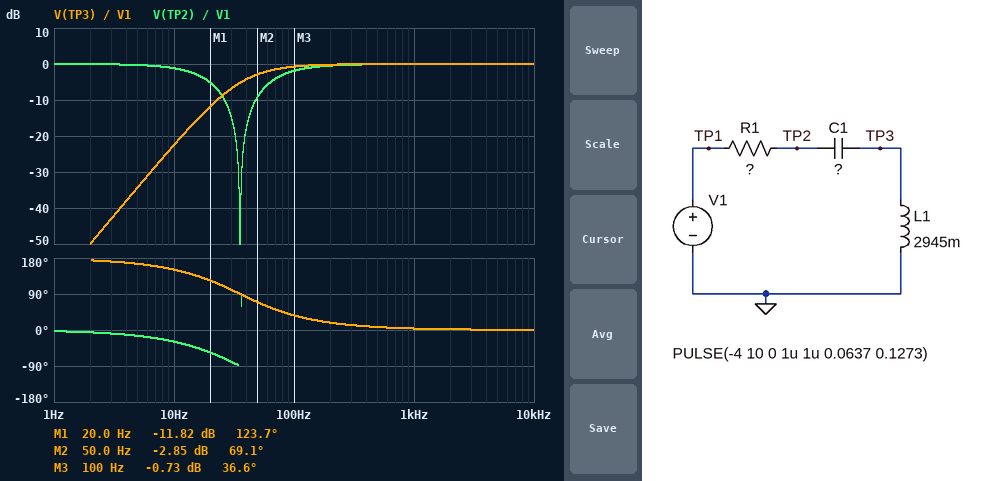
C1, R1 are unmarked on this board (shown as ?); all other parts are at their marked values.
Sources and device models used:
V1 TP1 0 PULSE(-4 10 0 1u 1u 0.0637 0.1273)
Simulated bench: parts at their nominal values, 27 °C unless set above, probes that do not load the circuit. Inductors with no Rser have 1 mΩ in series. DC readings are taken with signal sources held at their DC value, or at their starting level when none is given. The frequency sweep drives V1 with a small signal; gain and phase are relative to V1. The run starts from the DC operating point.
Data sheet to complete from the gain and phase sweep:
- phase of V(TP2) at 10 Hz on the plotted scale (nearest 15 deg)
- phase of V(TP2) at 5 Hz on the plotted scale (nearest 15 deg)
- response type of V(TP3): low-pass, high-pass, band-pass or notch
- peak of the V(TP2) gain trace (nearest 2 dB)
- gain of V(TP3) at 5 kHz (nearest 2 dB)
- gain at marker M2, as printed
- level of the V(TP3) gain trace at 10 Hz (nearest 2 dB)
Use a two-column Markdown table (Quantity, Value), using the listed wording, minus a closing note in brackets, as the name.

| Quantity | Value |
|---|---|
| phase of V(TP2) at 10 Hz on the plotted scale | -30 deg |
| phase of V(TP2) at 5 Hz on the plotted scale | -15 deg |
| response type of V(TP3): low-pass, high-pass, band-pass or notch | high-pass |
| peak of the V(TP2) gain trace | 0 dB |
| gain of V(TP3) at 5 kHz | 0 dB |
| gain at marker M2, as printed | -2.85 dB |
| level of the V(TP3) gain trace at 10 Hz | -22 dB |
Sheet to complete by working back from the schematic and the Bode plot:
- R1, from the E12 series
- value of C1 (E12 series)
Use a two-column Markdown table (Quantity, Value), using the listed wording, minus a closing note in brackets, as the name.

| Quantity | Value |
|---|---|
| R1, from the E12 series | 1.2 kΩ |
| value of C1 | 6.8 µF |
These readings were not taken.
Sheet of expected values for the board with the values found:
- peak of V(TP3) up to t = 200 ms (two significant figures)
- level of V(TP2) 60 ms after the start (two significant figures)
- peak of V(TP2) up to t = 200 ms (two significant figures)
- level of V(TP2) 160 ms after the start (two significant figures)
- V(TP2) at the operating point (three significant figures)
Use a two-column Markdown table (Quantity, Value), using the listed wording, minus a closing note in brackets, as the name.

| Quantity | Value |
|---|---|
| peak of V(TP3) up to t = 200 ms | 14 V |
| level of V(TP2) 60 ms after the start | 10 V |
| peak of V(TP2) up to t = 200 ms | 10 V |
| level of V(TP2) 160 ms after the start | 10 V |
| V(TP2) at the operating point | -4.00 V |
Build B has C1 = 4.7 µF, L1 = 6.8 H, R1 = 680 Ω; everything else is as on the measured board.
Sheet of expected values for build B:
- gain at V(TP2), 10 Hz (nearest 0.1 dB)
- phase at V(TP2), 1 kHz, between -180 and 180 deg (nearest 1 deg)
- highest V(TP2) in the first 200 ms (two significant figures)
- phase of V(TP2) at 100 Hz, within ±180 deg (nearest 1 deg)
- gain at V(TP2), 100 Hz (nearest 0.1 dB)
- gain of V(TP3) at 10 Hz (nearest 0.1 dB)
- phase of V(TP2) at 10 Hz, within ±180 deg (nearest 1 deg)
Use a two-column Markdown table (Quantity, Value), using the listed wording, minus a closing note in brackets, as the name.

| Quantity | Value |
|---|---|
| gain at V(TP2), 10 Hz | -0.2 dB |
| phase at V(TP2), 1 kHz, between -180 and 180 deg | 1 deg |
| highest V(TP2) in the first 200 ms | 12 V |
| phase of V(TP2) at 100 Hz, within ±180 deg | 10 deg |
| gain at V(TP2), 100 Hz | -0.1 dB |
| gain of V(TP3) at 10 Hz | -17.0 dB |
| phase of V(TP2) at 10 Hz, within ±180 deg | -13 deg |
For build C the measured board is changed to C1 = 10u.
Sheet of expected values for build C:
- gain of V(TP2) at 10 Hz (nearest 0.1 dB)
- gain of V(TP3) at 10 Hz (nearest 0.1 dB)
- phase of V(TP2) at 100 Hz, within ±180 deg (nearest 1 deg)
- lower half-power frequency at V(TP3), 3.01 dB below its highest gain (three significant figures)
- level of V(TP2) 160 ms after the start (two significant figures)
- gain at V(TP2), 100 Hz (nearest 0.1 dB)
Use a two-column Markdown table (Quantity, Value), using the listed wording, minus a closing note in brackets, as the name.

| Quantity | Value |
|---|---|
| gain of V(TP2) at 10 Hz | -2.4 dB |
| gain of V(TP3) at 10 Hz | -20.0 dB |
| phase of V(TP2) at 100 Hz, within ±180 deg | 35 deg |
| lower half-power frequency at V(TP3), 3.01 dB below its highest gain | 52.5 Hz |
| level of V(TP2) 160 ms after the start | 9.3 V |
| gain at V(TP2), 100 Hz | -1.8 dB |
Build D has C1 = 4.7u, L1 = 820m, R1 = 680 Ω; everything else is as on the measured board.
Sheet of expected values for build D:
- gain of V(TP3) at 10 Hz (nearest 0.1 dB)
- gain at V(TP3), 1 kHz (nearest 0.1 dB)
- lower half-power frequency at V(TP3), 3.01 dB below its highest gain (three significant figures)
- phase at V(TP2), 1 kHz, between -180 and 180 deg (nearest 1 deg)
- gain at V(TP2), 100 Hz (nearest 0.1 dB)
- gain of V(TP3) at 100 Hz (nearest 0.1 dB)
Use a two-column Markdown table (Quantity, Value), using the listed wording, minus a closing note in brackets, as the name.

| Quantity | Value |
|---|---|
| gain of V(TP3) at 10 Hz | -36.4 dB |
| gain at V(TP3), 1 kHz | 0 dB |
| lower half-power frequency at V(TP3), 3.01 dB below its highest gain | 95.1 Hz |
| phase at V(TP2), 1 kHz, between -180 and 180 deg | 8 deg |
| gain at V(TP2), 100 Hz | -12.0 dB |
| gain of V(TP3) at 100 Hz | -2.7 dB |
